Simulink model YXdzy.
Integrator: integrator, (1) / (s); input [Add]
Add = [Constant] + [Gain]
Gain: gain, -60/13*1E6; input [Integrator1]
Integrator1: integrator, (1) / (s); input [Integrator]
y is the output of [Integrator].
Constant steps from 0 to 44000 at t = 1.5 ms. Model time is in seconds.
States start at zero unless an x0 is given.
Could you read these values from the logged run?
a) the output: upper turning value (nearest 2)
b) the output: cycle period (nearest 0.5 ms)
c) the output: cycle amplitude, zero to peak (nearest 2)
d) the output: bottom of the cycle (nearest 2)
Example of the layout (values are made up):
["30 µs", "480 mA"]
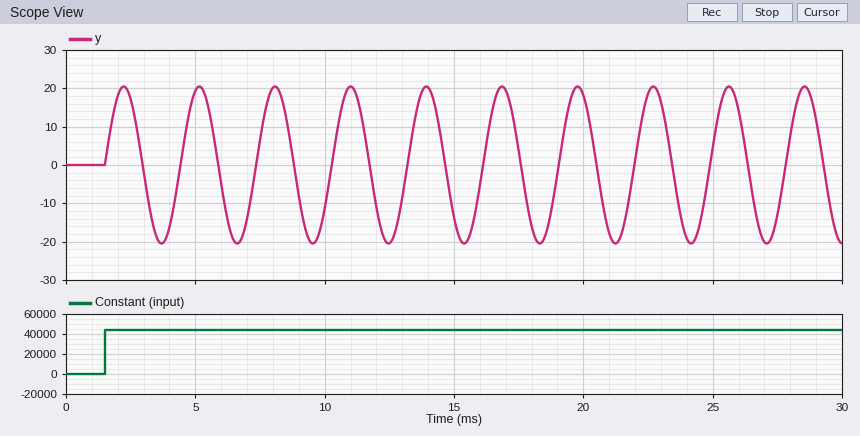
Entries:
["20", "3.0 ms", "20", "-20"]
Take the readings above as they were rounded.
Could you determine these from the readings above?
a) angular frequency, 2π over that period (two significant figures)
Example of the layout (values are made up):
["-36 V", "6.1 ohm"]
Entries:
["2.1 rad/ms"]
